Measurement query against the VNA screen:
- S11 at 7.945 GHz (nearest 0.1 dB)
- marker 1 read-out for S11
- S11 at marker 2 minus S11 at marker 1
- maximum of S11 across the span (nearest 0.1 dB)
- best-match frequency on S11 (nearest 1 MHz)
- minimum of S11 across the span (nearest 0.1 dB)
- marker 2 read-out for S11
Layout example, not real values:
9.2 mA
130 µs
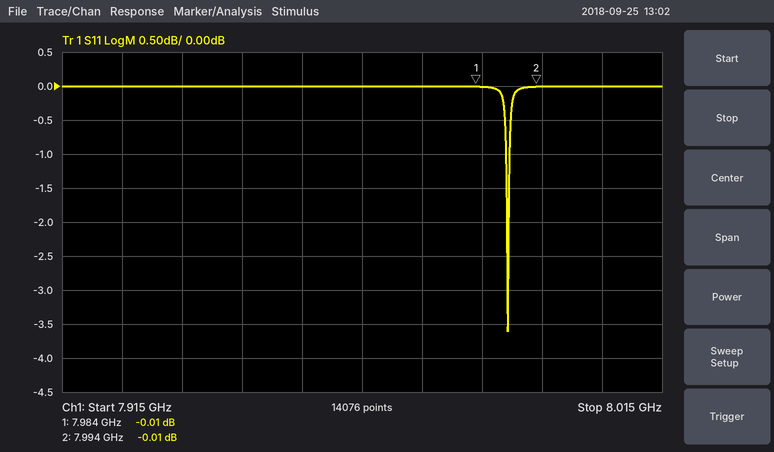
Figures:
0.0 dB
-0.01 dB
0.00 dB
0.0 dB
7.989 GHz
-3.6 dB
-0.01 dB
